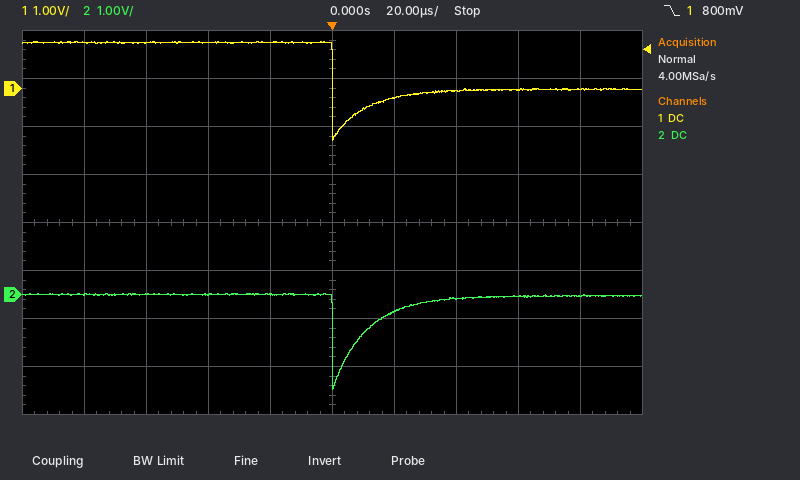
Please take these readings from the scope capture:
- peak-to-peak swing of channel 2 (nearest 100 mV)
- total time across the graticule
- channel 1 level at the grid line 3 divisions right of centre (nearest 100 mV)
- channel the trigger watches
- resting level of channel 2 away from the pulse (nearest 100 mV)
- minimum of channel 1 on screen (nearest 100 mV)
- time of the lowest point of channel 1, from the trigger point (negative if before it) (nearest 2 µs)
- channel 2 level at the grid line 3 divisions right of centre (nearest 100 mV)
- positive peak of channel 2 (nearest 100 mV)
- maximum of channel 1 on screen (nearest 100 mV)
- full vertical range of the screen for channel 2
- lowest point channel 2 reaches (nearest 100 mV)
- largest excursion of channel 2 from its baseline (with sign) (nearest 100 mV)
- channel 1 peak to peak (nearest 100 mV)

2.0 V
200 µs
0.0 V
channel 1
0.0 V
-1.1 V
0 µs
0.0 V
0.0 V
1.0 V
8 V
-2.0 V
-2.0 V
2.1 V
